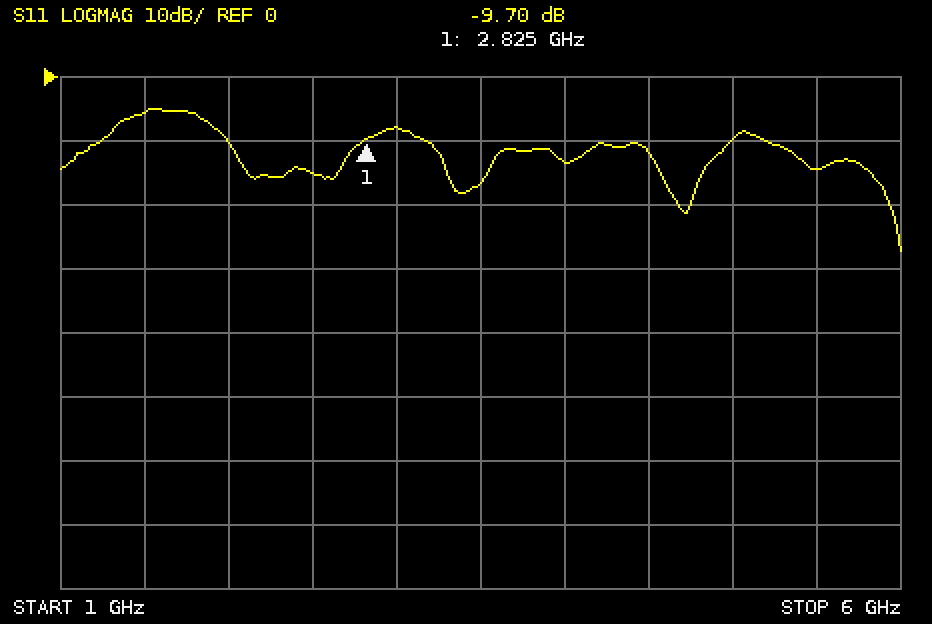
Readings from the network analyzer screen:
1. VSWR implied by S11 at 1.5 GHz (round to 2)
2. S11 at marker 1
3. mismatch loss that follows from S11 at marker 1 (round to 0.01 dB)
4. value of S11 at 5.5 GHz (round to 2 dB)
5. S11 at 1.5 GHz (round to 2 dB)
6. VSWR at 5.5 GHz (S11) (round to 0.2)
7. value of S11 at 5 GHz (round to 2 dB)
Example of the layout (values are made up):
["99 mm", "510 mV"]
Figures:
["4", "-9.70 dB", "0.49 dB", "-14 dB", "-6 dB", "1.4", "-10 dB"]
